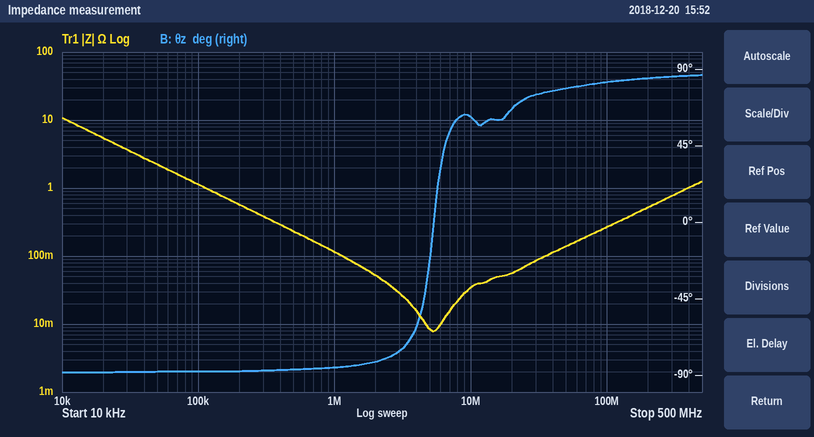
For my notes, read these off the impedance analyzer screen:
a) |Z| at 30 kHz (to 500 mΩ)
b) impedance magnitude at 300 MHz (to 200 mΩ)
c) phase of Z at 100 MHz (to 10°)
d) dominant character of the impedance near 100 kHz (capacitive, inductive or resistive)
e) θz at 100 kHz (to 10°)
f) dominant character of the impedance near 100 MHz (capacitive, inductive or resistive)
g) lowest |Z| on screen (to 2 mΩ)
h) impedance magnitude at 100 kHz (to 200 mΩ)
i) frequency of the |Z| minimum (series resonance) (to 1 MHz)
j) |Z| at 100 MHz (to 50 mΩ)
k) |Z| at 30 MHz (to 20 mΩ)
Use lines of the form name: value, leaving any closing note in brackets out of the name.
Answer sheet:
|Z| at 30 kHz: 3.5 Ω
impedance magnitude at 300 MHz: 800 mΩ
phase of Z at 100 MHz: 80°
dominant character of the impedance near 100 kHz: capacitive
θz at 100 kHz: -90°
dominant character of the impedance near 100 MHz: inductive
lowest |Z| on screen: 8 mΩ
impedance magnitude at 100 kHz: 1.2 Ω
frequency of the |Z| minimum (series resonance): 5 MHz
|Z| at 100 MHz: 250 mΩ
|Z| at 30 MHz: 80 mΩ
